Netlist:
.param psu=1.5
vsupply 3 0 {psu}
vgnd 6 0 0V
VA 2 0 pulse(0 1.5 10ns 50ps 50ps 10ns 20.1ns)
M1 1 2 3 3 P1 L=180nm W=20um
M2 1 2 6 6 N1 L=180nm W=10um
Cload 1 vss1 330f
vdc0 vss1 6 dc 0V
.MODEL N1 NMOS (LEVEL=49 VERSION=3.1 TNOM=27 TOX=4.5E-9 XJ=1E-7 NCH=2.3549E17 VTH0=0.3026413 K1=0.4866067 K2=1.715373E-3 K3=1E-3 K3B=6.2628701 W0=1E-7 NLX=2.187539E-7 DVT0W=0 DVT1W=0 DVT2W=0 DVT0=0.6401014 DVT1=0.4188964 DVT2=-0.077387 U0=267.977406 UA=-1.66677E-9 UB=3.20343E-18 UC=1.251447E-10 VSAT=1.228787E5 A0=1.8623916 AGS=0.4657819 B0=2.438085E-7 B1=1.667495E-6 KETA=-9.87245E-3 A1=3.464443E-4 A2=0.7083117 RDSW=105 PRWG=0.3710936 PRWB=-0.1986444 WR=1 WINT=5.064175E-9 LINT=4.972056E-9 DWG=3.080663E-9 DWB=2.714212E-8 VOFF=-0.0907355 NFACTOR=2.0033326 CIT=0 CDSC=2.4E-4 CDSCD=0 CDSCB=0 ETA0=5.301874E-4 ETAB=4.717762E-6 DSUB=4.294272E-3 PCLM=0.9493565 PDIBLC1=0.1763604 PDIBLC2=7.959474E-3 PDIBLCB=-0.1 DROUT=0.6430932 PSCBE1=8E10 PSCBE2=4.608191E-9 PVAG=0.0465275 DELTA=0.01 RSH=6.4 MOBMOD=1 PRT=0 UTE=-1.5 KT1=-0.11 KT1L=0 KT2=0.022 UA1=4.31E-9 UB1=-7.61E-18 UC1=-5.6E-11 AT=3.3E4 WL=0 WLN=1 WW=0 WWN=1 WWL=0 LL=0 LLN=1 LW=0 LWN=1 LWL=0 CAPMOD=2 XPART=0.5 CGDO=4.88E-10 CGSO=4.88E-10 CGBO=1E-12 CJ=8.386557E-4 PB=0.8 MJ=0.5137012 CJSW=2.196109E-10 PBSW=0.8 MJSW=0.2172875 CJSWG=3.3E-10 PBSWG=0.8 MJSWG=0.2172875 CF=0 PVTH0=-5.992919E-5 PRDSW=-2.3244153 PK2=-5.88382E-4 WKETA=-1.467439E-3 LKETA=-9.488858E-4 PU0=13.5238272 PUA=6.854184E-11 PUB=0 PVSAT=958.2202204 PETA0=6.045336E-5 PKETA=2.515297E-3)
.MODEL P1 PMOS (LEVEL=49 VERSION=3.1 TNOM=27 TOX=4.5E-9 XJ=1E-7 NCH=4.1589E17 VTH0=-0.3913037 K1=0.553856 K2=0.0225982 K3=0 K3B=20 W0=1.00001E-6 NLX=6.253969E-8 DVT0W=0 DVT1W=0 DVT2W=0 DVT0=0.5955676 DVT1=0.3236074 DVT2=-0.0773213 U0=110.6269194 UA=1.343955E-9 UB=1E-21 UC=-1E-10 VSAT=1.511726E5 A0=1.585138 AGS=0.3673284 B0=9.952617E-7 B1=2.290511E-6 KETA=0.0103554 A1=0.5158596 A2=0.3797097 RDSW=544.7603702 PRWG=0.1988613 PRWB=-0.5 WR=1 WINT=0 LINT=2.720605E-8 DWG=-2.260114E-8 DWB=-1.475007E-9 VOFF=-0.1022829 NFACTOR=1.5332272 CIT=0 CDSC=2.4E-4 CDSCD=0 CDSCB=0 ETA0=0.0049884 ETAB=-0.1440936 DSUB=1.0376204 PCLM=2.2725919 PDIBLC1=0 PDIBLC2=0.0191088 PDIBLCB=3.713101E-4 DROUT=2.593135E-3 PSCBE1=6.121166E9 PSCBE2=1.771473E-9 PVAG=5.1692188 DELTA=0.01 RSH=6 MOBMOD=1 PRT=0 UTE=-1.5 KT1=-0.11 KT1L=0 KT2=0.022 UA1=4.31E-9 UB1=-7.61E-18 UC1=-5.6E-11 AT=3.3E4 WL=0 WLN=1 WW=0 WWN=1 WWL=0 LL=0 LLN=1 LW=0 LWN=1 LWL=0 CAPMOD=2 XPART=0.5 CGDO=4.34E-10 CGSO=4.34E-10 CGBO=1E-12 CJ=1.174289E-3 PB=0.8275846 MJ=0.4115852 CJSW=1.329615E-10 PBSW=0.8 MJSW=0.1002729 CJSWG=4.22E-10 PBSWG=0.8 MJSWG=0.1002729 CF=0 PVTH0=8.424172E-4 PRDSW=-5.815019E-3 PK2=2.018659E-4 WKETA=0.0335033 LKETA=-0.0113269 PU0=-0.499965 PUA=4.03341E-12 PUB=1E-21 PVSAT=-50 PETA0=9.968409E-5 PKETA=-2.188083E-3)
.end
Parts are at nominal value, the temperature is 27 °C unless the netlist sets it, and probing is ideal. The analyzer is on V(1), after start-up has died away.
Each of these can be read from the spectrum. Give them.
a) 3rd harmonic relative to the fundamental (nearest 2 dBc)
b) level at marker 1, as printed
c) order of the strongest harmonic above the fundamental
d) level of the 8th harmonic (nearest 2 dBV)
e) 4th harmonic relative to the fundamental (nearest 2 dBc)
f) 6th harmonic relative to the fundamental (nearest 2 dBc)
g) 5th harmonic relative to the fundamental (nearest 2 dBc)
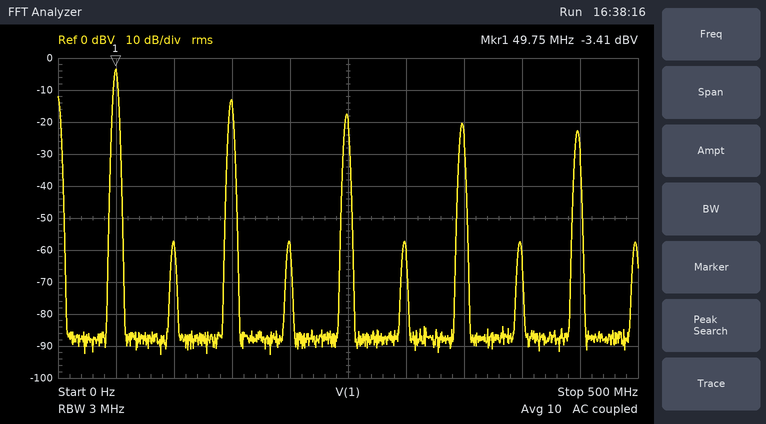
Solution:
-10 dBc
-3.41 dBV
3
-58 dBV
-54 dBc
-54 dBc
-14 dBc
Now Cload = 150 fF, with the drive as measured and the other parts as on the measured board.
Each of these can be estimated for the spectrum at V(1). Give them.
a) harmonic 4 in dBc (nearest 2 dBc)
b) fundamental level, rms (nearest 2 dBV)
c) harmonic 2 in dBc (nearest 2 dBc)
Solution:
-60 dBc
-4 dBV
-60 dBc
